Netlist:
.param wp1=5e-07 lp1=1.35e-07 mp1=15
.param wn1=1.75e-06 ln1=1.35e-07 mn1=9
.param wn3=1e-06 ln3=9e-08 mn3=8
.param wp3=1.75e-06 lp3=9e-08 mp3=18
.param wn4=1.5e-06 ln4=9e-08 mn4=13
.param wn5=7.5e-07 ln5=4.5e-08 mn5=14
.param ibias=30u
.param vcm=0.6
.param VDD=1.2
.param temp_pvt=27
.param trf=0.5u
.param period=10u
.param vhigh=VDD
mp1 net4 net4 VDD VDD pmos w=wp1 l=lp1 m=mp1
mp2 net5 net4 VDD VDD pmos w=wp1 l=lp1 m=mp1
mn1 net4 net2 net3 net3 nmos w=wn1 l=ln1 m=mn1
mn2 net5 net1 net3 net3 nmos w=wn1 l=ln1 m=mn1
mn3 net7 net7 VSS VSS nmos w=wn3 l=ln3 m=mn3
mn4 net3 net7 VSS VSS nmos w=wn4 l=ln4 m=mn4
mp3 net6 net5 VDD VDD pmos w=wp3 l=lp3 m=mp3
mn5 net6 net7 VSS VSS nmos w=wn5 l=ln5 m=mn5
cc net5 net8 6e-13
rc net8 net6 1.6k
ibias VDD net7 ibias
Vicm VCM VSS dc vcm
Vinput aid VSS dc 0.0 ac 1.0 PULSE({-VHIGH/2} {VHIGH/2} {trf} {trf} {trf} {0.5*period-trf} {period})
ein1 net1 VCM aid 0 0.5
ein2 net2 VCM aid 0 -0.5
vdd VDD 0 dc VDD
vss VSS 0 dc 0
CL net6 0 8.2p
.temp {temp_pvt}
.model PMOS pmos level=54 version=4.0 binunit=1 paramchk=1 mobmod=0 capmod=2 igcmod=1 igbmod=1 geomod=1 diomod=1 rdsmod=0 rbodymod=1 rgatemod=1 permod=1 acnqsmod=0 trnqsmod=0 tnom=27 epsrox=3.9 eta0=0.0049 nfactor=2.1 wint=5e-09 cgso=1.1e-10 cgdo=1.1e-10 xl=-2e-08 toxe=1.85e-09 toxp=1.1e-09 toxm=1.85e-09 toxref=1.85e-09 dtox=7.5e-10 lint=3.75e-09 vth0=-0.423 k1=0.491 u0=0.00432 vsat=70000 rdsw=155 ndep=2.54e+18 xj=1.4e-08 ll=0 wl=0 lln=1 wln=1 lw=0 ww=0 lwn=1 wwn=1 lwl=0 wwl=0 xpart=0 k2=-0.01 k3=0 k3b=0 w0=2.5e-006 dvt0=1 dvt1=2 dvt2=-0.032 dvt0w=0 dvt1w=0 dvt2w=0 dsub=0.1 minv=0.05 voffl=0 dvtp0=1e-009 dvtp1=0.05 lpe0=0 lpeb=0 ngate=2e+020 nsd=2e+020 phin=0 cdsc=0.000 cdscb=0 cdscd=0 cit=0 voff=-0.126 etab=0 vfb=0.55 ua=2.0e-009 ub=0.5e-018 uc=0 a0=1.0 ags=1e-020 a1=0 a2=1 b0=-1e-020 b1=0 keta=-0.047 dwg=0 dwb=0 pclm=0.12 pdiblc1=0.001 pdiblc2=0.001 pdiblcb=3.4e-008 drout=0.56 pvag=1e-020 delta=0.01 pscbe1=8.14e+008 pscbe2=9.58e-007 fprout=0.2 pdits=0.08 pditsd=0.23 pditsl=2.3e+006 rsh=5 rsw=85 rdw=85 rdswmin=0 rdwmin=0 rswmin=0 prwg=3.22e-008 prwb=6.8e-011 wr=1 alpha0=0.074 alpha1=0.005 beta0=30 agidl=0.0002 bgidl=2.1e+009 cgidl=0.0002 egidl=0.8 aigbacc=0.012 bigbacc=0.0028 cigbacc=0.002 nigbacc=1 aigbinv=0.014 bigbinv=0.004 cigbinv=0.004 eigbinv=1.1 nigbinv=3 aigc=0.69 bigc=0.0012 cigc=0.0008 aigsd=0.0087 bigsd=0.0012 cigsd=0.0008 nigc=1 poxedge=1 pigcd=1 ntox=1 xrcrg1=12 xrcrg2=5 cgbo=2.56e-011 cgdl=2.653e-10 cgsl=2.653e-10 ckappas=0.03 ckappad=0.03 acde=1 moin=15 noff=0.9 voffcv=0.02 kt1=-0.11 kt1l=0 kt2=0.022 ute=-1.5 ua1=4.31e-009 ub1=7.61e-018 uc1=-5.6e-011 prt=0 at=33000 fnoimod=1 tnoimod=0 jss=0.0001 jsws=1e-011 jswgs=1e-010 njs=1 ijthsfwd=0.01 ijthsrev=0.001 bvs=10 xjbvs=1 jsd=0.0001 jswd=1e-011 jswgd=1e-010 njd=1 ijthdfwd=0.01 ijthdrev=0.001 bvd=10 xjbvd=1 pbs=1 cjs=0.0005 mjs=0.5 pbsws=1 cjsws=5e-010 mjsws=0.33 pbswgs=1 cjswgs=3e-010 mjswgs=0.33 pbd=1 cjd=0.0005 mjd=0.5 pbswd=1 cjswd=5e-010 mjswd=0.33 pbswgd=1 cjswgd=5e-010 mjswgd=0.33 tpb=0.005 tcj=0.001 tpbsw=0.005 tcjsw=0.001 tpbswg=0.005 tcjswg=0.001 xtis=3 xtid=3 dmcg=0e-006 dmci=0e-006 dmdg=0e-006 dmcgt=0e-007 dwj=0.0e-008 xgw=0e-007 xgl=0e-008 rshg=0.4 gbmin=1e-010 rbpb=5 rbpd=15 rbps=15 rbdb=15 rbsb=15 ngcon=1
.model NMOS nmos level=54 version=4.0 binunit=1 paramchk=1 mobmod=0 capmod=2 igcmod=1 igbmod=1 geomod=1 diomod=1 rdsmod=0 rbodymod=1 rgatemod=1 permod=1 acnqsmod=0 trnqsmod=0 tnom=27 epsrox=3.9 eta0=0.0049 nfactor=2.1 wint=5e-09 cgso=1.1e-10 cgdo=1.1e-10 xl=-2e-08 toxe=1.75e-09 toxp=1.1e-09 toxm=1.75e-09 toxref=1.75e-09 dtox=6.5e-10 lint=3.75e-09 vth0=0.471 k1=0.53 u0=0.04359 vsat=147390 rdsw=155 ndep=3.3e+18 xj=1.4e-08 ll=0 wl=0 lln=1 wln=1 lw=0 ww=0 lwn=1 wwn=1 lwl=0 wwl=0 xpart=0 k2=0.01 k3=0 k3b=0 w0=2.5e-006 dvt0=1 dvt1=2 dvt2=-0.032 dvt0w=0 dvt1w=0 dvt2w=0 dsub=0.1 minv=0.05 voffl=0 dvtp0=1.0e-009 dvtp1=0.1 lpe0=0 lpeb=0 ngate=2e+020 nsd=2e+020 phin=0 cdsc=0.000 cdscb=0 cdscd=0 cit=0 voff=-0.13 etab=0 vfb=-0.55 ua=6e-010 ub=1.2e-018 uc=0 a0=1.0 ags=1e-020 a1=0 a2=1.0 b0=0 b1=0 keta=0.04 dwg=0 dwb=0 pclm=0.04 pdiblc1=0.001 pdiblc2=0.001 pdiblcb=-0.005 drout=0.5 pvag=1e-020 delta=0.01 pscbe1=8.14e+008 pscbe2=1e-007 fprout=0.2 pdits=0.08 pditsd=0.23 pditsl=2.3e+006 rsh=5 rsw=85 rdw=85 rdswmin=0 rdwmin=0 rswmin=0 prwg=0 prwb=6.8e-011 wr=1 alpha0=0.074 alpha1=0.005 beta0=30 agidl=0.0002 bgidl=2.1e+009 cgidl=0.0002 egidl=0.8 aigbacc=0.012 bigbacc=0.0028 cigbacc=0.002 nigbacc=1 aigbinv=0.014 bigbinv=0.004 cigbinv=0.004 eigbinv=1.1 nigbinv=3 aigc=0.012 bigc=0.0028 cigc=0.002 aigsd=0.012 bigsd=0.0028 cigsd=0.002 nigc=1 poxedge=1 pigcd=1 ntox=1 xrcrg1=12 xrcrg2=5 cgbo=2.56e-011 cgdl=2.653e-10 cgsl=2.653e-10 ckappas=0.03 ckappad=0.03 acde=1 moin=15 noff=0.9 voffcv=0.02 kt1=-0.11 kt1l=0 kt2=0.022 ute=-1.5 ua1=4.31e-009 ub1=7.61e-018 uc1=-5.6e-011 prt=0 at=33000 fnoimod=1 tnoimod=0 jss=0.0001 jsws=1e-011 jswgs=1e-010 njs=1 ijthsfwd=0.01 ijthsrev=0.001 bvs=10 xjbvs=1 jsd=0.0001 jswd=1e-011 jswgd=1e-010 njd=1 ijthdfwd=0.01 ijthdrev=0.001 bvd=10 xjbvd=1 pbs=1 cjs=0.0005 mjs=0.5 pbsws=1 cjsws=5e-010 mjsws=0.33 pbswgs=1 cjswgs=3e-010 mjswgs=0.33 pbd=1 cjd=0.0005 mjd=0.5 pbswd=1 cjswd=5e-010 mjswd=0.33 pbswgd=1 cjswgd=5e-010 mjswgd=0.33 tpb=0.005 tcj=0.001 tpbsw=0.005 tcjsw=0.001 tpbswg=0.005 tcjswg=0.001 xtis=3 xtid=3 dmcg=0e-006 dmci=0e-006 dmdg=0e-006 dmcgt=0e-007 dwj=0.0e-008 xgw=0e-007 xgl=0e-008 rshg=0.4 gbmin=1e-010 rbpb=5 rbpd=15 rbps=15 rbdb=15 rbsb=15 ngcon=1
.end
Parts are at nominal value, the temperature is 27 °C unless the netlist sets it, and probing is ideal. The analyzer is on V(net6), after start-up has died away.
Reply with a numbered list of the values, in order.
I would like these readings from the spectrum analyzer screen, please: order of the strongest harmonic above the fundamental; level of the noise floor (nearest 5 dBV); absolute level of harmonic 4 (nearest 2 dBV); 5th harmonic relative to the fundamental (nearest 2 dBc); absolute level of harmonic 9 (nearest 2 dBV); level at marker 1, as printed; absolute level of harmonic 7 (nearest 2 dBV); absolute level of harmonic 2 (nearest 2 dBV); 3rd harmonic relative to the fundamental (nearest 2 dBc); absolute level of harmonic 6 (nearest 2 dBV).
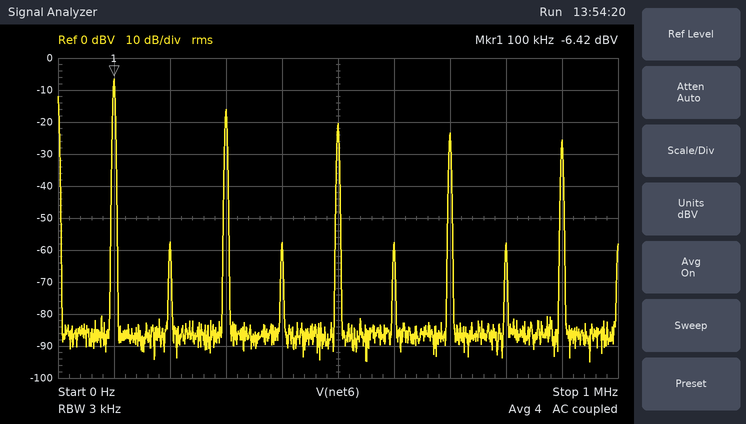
1. 3
2. -85 dBV
3. -58 dBV
4. -14 dBc
5. -26 dBV
6. -6.42 dBV
7. -24 dBV
8. -58 dBV
9. -10 dBc
10. -58 dBV
